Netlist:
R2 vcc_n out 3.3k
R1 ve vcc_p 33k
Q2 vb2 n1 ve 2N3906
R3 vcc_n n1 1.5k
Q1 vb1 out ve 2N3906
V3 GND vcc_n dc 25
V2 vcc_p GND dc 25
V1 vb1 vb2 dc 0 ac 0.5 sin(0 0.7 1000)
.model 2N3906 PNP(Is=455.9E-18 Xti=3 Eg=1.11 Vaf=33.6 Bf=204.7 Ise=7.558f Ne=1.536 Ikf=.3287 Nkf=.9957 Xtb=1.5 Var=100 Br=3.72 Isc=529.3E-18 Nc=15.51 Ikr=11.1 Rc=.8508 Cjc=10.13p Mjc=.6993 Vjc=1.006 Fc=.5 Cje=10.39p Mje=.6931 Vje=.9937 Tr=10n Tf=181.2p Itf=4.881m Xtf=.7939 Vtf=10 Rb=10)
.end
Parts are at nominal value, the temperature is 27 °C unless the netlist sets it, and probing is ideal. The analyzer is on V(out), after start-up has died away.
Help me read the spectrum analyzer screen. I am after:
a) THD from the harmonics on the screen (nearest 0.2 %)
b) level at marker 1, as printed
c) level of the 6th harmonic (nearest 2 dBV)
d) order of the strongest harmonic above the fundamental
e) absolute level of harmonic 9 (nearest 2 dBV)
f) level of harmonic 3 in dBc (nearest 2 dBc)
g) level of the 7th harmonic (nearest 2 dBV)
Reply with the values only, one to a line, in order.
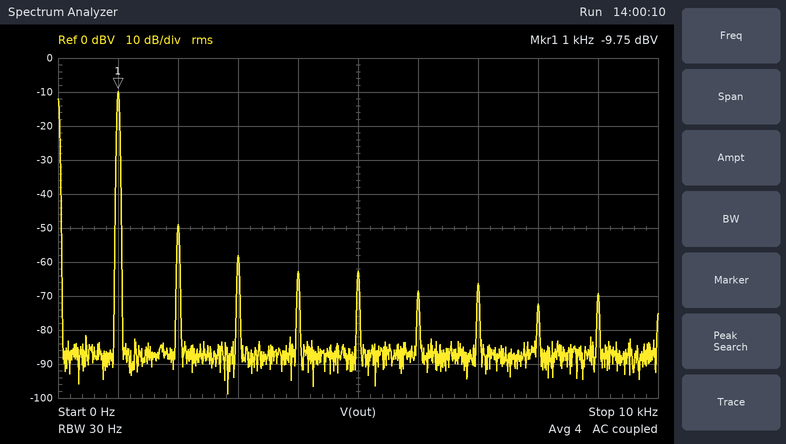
1.2 %
-9.75 dBV
-68 dBV
2
-70 dBV
-48 dBc
-66 dBV
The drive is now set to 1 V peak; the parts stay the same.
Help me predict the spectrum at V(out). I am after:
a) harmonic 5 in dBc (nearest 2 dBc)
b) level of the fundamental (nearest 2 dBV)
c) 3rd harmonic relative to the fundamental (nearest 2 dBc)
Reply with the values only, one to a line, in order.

-56 dBc
-6 dBV
-52 dBc
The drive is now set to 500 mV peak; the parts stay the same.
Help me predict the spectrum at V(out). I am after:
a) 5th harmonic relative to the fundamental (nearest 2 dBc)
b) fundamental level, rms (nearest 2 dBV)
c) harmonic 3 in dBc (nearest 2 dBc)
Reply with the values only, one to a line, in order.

-50 dBc
-12 dBV
-46 dBc
